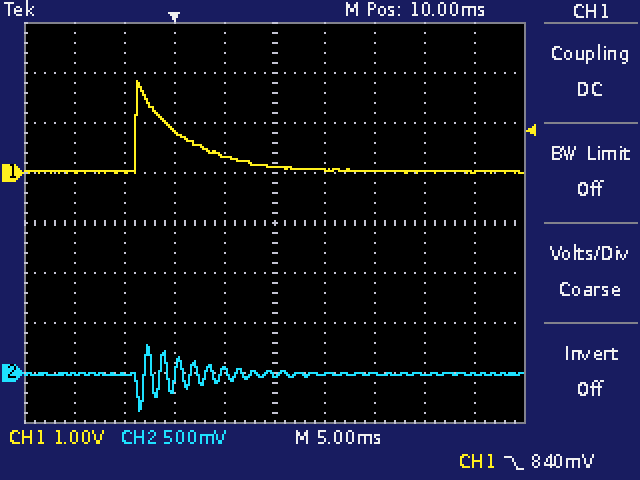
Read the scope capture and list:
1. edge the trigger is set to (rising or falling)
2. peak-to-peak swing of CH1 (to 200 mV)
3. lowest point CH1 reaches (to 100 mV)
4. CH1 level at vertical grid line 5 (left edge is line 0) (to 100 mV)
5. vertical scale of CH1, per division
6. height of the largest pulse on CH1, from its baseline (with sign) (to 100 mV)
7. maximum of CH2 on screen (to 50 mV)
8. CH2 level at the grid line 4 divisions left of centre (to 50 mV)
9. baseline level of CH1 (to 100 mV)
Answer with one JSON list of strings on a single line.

["falling", "1.8 V", "0.0 V", "100 mV", "1 V", "+1.8 V", "300 mV", "0 mV", "0.0 V"]
